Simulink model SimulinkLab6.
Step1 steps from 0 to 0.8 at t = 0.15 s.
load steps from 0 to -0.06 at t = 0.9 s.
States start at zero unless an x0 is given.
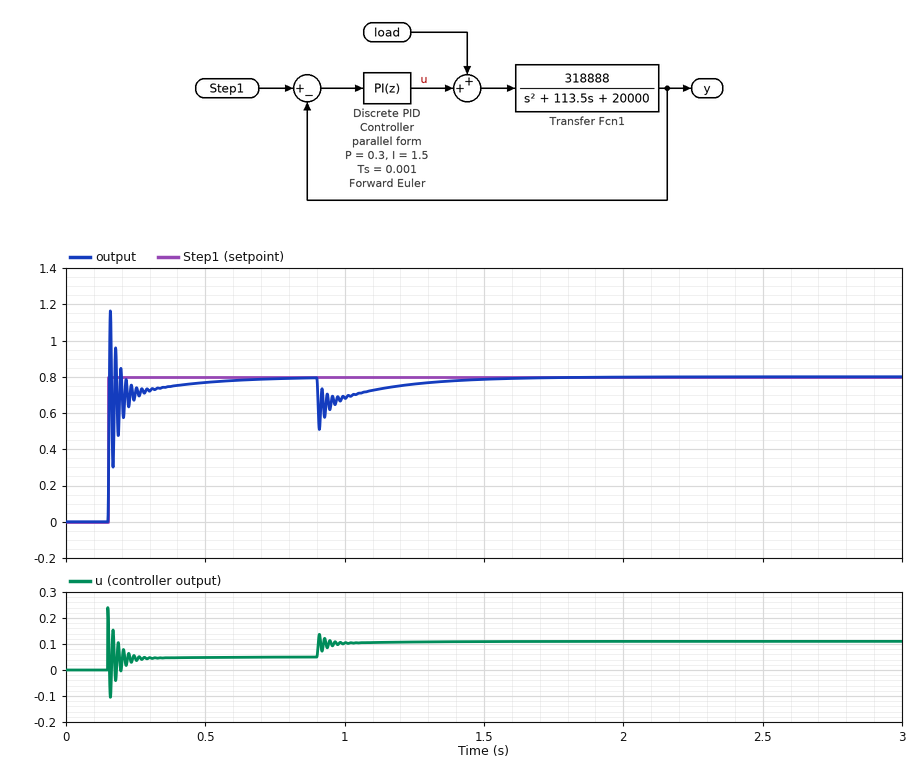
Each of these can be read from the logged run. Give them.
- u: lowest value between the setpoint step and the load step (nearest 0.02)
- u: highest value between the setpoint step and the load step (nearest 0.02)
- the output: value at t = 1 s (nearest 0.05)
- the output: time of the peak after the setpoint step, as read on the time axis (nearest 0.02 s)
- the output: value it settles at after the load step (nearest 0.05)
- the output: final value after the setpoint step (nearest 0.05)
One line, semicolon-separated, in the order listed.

-0.10; 0.24; 0.70; 0.16 s; 0.80; 0.80
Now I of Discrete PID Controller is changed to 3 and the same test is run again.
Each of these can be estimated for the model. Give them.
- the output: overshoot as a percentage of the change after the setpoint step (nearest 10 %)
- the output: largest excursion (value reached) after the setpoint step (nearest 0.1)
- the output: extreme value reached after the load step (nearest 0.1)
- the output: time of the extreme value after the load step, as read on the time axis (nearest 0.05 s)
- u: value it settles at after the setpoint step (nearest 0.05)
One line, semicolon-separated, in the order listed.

50 %; 1.2; 0.5; 0.90 s; 0.05
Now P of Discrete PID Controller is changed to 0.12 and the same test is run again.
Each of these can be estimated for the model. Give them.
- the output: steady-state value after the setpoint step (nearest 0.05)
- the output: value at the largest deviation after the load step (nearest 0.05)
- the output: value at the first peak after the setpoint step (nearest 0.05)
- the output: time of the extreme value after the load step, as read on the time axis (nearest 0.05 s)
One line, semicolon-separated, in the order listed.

0.80; 0.30; 0.85; 0.90 s
